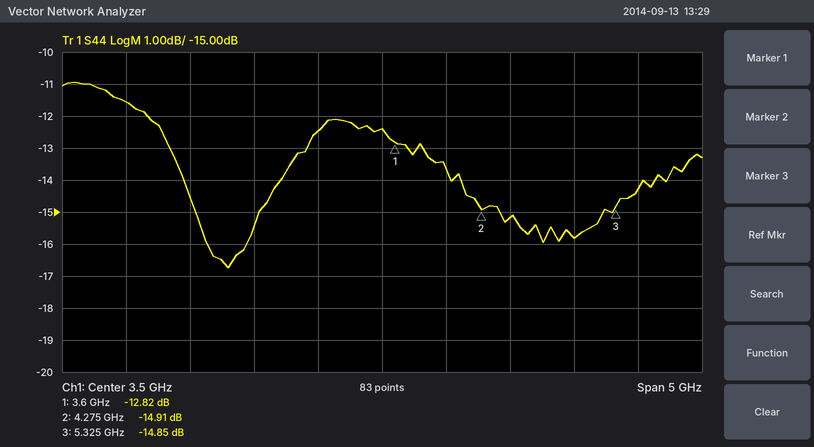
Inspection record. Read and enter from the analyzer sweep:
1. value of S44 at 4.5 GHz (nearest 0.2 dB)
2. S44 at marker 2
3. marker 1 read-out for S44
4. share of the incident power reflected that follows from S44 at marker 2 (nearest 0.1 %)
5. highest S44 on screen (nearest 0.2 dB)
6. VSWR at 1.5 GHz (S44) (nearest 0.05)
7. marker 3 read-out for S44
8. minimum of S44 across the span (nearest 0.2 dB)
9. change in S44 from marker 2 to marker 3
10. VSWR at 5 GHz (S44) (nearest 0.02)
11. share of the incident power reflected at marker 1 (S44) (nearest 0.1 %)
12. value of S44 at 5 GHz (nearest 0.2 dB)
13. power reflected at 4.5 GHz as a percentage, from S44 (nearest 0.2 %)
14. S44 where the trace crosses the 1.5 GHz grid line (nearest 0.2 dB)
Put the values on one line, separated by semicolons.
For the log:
-15.2 dB; -14.91 dB; -12.82 dB; 3.2 %; -11.0 dB; 1.70; -14.85 dB; -16.8 dB; 0.06 dB; 1.38; 5.2 %; -15.8 dB; 3.0 %; -11.6 dB
